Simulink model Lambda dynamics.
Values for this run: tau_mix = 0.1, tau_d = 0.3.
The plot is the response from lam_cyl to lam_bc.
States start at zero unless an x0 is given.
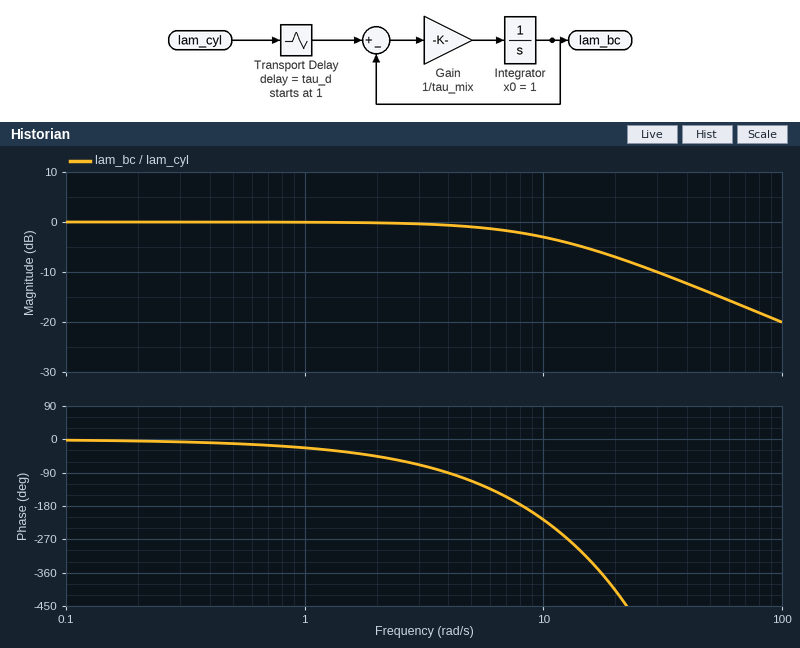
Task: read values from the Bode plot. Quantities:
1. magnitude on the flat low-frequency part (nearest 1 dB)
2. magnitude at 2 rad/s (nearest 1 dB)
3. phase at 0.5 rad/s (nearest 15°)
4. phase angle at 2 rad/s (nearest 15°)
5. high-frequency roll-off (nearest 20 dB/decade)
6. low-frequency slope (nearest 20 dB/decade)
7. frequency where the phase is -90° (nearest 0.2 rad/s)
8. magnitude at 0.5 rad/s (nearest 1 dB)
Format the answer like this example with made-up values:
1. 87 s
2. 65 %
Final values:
1. 0 dB
2. 0 dB
3. -15°
4. -45°
5. -20 dB/decade
6. 0 dB/decade
7. 4.0 rad/s
8. 0 dB
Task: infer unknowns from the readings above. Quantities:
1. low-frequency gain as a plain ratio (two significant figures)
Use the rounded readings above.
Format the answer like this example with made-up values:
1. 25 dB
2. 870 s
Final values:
1. 1.0
